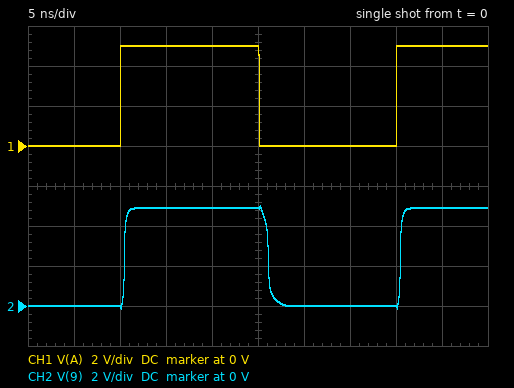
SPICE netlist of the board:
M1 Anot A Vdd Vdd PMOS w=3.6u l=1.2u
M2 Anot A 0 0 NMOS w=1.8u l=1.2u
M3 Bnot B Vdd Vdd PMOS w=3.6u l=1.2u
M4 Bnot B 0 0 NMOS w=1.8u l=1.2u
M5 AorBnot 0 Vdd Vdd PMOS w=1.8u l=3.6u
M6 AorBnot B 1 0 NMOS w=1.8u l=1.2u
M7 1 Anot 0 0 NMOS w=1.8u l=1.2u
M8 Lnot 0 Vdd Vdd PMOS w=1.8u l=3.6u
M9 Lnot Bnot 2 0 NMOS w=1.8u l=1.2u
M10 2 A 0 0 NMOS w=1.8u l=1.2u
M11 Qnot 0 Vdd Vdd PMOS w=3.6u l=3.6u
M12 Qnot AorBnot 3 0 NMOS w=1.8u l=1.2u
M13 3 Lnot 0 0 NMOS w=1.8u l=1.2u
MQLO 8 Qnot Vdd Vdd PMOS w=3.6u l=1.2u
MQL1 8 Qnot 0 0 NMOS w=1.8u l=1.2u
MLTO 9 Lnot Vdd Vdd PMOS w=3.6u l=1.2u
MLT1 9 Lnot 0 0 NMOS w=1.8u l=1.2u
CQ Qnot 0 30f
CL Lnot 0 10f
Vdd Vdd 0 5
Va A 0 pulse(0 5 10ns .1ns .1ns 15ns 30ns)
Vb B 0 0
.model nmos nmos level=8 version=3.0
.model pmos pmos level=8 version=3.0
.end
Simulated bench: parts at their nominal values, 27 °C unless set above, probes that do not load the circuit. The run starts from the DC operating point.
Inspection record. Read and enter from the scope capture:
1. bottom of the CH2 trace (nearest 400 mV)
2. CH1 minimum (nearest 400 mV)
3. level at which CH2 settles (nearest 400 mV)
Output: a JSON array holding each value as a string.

["0 V", "0 V", "4.8 V"]
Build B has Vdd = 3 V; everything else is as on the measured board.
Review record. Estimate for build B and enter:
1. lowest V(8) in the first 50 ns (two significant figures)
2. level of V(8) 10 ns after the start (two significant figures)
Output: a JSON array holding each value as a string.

["-16 mV", "2.9 V"]
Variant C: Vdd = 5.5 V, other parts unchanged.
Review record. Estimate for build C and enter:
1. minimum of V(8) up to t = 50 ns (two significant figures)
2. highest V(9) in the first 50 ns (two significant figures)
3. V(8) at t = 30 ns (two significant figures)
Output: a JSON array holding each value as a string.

["3.9 mV", "5.4 V", "4.9 V"]
